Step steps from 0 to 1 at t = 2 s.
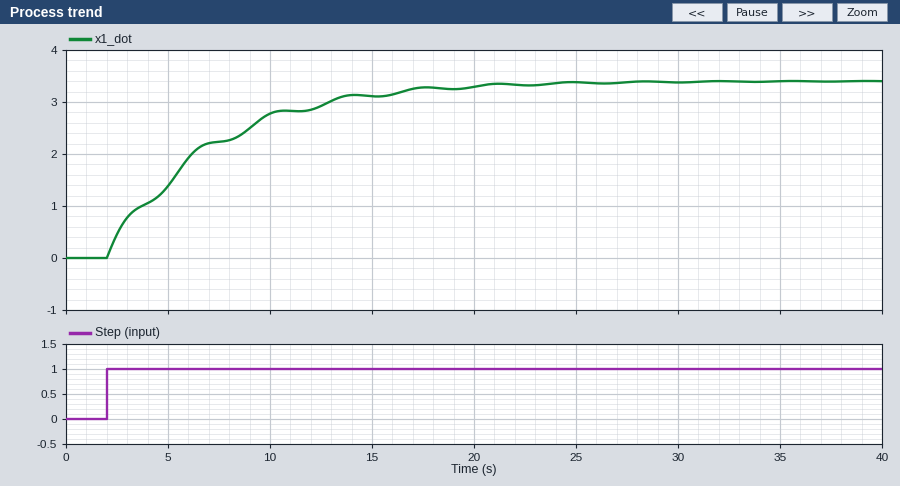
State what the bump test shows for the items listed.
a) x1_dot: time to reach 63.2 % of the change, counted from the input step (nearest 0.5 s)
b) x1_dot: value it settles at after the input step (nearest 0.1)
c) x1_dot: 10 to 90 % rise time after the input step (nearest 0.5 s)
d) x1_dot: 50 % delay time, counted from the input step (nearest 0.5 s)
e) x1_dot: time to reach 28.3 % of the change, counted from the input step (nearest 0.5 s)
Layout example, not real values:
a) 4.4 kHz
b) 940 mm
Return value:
a) 4.5 s
b) 3.4
c) 11.0 s
d) 3.5 s
e) 1.5 s
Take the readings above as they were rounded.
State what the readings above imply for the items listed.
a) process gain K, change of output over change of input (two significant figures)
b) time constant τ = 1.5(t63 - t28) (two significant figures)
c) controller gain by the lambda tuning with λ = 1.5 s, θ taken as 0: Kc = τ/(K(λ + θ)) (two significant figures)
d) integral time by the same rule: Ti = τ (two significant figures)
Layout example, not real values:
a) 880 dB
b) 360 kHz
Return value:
a) 3.4
b) 4.5 s
c) 0.88
d) 4.5 s
